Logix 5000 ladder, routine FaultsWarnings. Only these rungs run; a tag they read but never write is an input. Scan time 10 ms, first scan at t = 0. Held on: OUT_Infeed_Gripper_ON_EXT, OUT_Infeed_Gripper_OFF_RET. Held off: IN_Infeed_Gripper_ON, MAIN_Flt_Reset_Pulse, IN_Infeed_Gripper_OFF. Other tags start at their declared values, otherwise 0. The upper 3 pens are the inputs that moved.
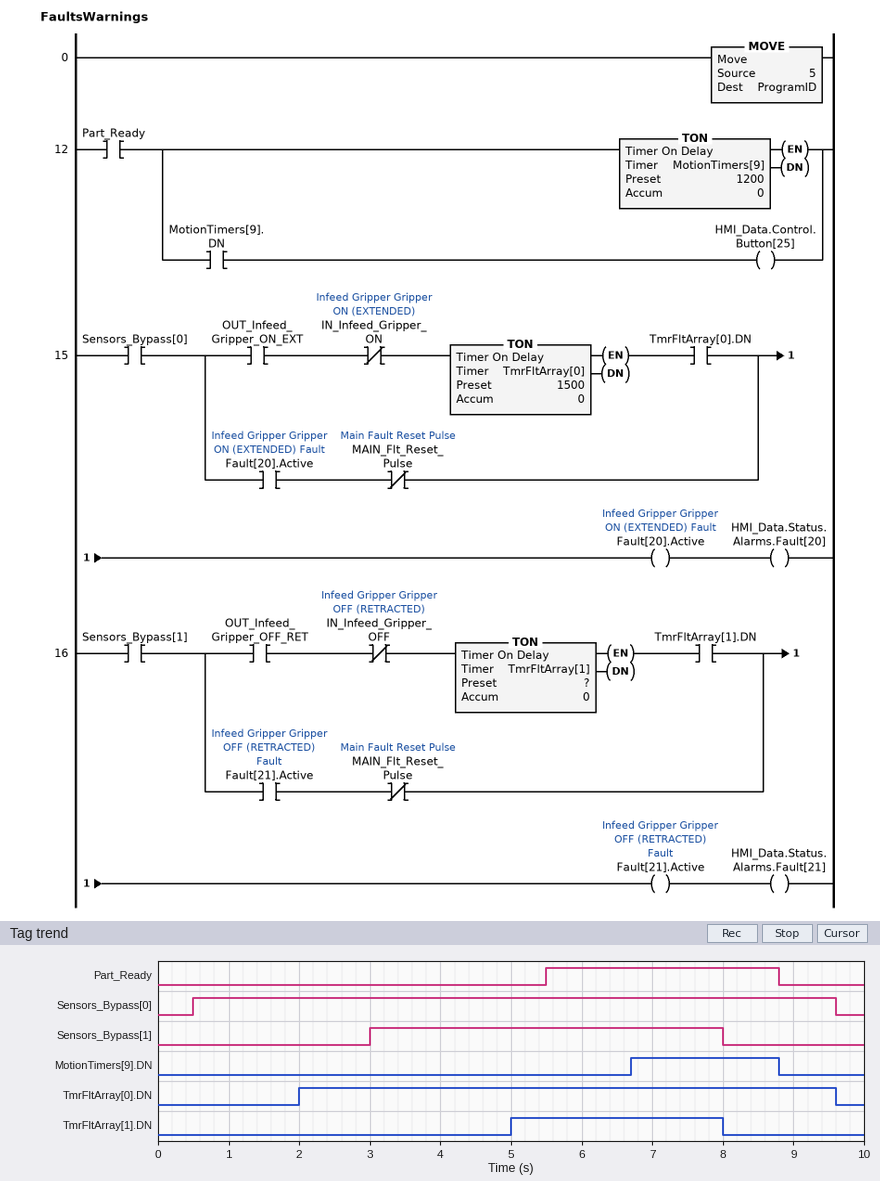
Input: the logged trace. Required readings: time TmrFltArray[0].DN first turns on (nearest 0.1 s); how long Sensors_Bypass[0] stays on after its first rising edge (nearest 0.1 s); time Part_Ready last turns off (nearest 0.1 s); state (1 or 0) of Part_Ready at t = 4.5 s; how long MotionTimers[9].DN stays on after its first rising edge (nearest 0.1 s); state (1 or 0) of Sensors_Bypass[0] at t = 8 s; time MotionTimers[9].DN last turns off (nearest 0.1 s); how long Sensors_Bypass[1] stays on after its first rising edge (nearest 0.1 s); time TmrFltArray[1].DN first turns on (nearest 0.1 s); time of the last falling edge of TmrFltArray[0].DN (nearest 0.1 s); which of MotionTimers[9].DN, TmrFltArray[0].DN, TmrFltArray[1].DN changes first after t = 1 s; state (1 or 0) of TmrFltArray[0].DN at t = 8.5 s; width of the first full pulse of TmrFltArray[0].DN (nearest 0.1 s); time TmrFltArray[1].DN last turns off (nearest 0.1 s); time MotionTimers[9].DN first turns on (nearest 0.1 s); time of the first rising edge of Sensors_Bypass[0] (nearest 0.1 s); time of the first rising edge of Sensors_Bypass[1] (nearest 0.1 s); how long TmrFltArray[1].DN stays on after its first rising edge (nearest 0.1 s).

2.0 s
9.1 s
8.8 s
0
2.1 s
1
8.8 s
5.0 s
5.0 s
9.6 s
TmrFltArray[0].DN
1
7.6 s
8.0 s
6.7 s
0.5 s
3.0 s
3.0 s
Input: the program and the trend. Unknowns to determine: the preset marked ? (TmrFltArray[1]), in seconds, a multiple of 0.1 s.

2.0 s
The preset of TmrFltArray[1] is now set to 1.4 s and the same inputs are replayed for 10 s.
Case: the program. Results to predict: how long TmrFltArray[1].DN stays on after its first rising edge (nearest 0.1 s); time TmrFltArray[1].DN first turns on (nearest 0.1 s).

3.6 s
4.4 s
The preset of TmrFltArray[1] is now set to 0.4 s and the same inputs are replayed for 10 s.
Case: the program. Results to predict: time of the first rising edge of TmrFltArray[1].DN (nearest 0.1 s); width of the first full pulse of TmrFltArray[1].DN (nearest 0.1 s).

3.4 s
4.6 s
